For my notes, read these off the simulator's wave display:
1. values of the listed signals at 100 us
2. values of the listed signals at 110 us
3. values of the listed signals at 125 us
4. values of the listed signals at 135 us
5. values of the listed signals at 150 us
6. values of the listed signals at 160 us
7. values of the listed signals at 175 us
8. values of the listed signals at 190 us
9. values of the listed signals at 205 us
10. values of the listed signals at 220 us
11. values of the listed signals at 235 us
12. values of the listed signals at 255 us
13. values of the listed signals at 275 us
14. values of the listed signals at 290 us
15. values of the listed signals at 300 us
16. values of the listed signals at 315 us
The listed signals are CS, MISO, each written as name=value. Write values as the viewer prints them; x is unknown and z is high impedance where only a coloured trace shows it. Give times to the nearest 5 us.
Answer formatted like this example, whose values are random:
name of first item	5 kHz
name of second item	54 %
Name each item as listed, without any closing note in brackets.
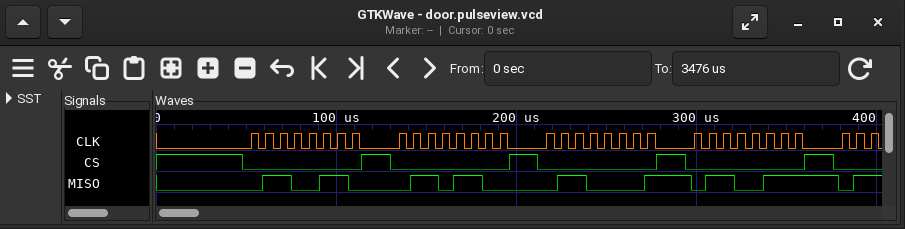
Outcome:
values of the listed signals at 100 us	CS=0, MISO=1
values of the listed signals at 110 us	CS=0, MISO=0
values of the listed signals at 125 us	CS=1, MISO=0
values of the listed signals at 135 us	CS=0, MISO=0
values of the listed signals at 150 us	CS=0, MISO=1
values of the listed signals at 160 us	CS=0, MISO=0
values of the listed signals at 175 us	CS=0, MISO=1
values of the listed signals at 190 us	CS=0, MISO=0
values of the listed signals at 205 us	CS=1, MISO=0
values of the listed signals at 220 us	CS=0, MISO=0
values of the listed signals at 235 us	CS=0, MISO=1
values of the listed signals at 255 us	CS=0, MISO=0
values of the listed signals at 275 us	CS=0, MISO=1
values of the listed signals at 290 us	CS=1, MISO=1
values of the listed signals at 300 us	CS=0, MISO=0
values of the listed signals at 315 us	CS=0, MISO=1
